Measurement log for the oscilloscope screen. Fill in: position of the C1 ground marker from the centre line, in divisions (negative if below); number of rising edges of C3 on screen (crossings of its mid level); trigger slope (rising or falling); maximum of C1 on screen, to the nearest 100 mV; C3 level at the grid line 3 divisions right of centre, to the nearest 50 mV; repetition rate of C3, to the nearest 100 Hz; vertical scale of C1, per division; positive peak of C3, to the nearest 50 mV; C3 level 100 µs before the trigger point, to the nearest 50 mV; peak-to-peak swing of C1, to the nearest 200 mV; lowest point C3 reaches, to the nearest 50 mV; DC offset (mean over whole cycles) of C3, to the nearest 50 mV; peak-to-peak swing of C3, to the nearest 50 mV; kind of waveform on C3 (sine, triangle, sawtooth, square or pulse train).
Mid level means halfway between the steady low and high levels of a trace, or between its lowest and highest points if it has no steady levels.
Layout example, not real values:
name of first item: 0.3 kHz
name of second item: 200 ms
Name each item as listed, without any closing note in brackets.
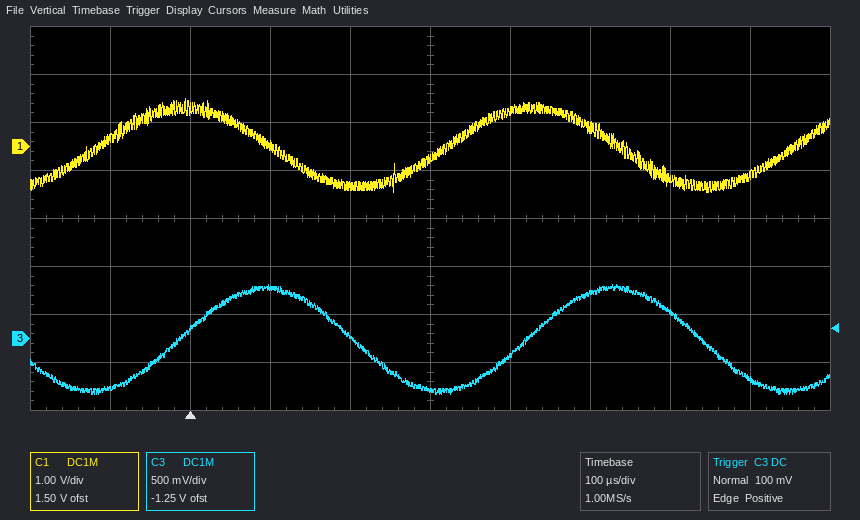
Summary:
position of the C1 ground marker from the centre line, in divisions: +1.5 div
number of rising edges of C3 on screen: 2
trigger slope: rising
maximum of C1 on screen, to the nearest 100 mV: 1.0 V
C3 level at the grid line 3 divisions right of centre, to the nearest 50 mV: 300 mV
repetition rate of C3, to the nearest 100 Hz: 2.3 kHz
vertical scale of C1, per division: 1 V
positive peak of C3, to the nearest 50 mV: 550 mV
C3 level 100 µs before the trigger point, to the nearest 50 mV: -500 mV
peak-to-peak swing of C1, to the nearest 200 mV: 2.0 V
lowest point C3 reaches, to the nearest 50 mV: -600 mV
DC offset (mean over whole cycles) of C3, to the nearest 50 mV: 0 mV
peak-to-peak swing of C3, to the nearest 50 mV: 1.15 V
kind of waveform on C3: sine
